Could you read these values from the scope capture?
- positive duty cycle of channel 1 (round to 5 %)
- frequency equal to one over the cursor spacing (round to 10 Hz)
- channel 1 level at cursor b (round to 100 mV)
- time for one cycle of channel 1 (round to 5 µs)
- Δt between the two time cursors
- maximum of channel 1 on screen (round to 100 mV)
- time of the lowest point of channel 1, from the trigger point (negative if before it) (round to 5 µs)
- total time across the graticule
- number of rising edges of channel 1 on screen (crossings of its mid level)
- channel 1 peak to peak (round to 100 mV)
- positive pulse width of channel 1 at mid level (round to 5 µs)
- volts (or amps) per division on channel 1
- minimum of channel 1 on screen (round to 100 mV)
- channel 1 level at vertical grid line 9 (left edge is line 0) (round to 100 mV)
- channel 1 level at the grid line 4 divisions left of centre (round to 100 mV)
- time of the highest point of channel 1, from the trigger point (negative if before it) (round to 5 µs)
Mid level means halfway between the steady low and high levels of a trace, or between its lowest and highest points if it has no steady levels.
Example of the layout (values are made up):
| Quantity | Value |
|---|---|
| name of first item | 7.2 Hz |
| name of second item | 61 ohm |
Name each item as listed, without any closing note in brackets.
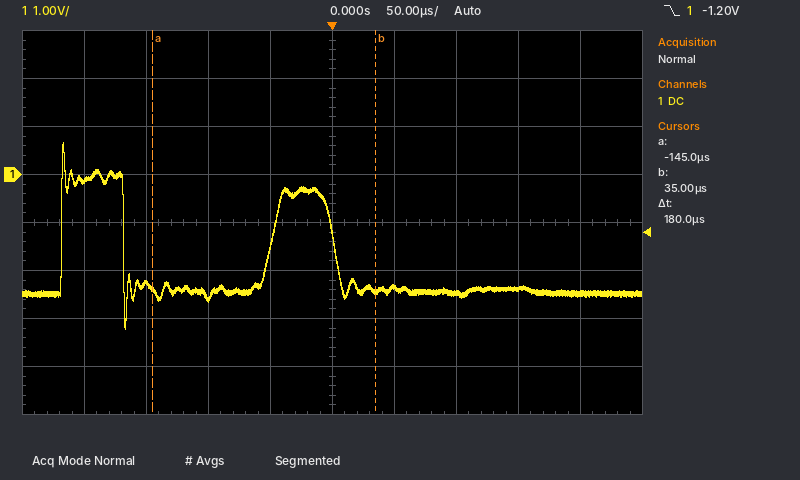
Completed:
| Quantity | Value |
|---|---|
| positive duty cycle of channel 1 | 30 % |
| frequency equal to one over the cursor spacing | 5.56 kHz |
| channel 1 level at cursor b | -2.4 V |
| time for one cycle of channel 1 | 170 µs |
| Δt between the two time cursors | 180 µs |
| maximum of channel 1 on screen | 700 mV |
| time of the lowest point of channel 1, from the trigger point (negative if before it) | -165 µs |
| total time across the graticule | 500 µs |
| number of rising edges of channel 1 on screen | 2 |
| channel 1 peak to peak | 3.9 V |
| positive pulse width of channel 1 at mid level | 50 µs |
| volts (or amps) per division on channel 1 | 1 V |
| minimum of channel 1 on screen | -3.2 V |
| channel 1 level at vertical grid line 9 (left edge is line 0) | -2.5 V |
| channel 1 level at the grid line 4 divisions left of centre | -100 mV |
| time of the highest point of channel 1, from the trigger point (negative if before it) | -215 µs |
